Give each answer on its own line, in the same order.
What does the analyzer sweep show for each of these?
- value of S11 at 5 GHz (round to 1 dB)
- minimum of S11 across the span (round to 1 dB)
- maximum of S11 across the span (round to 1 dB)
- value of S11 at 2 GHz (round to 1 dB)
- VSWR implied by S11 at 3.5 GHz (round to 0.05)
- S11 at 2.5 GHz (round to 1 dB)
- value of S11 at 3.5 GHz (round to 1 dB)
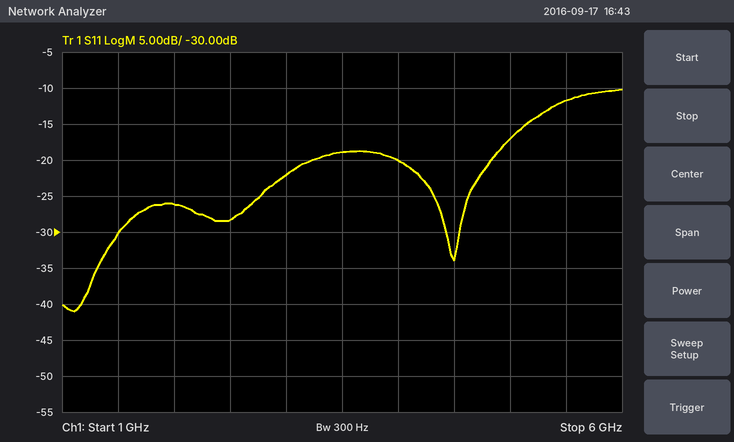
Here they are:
-17 dB
-41 dB
-10 dB
-26 dB
1.25
-28 dB
-19 dB
